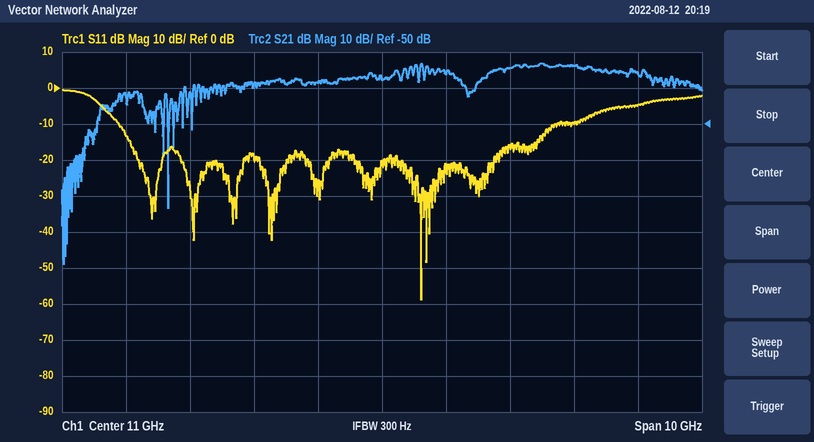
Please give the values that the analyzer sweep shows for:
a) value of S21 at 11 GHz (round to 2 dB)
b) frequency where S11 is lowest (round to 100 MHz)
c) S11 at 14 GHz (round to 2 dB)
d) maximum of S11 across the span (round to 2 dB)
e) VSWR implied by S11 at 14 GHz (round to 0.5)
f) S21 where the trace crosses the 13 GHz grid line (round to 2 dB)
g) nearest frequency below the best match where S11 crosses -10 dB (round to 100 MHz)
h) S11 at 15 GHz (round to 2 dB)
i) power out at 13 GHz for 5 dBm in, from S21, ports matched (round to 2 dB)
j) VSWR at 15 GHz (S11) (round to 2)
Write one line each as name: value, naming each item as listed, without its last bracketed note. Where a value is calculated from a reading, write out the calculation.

value of S21 at 11 GHz: -38 dB
frequency where S11 is lowest: 11.6 GHz
S11 at 14 GHz: -10 dB
maximum of S11 across the span: 0 dB
VSWR implied by S11 at 14 GHz: |Γ| = 10^(-10/20) = 0.3162; VSWR = (1 + 0.3162)/(1 − 0.3162) ≈ 1.92, so 2.0 to the nearest 0.5
S21 where the trace crosses the 13 GHz grid line: -34 dB
nearest frequency below the best match where S11 crosses -10 dB: 6.9 GHz
S11 at 15 GHz: -4 dB
power out at 13 GHz for 5 dBm in, from S21, ports matched: 5 dBm + (-34 dB) = -30 dBm
VSWR at 15 GHz (S11): |Γ| = 10^(-4/20) = 0.6310; VSWR = (1 + 0.6310)/(1 − 0.6310) ≈ 4
